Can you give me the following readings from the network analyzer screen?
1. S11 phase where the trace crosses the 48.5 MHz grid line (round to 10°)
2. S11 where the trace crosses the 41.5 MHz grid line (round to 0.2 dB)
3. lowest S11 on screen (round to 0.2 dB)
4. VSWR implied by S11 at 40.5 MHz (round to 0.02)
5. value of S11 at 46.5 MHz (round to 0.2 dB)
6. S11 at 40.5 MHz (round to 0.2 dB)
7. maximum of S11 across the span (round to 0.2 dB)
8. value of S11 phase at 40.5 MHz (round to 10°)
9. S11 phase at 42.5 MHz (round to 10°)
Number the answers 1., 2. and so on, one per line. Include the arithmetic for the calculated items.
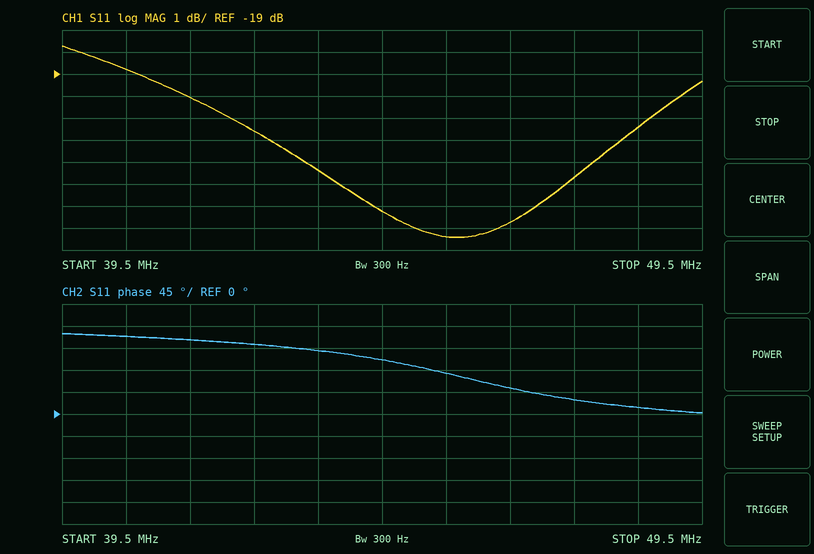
1. 10°
2. -20.0 dB
3. -26.4 dB
4. |Γ| = 10^(-18.8/20) = 0.1148; VSWR = (1 + 0.1148)/(1 − 0.1148) ≈ 1.26
5. -25.8 dB
6. -18.8 dB
7. -17.8 dB
8. 160°
9. 140°
